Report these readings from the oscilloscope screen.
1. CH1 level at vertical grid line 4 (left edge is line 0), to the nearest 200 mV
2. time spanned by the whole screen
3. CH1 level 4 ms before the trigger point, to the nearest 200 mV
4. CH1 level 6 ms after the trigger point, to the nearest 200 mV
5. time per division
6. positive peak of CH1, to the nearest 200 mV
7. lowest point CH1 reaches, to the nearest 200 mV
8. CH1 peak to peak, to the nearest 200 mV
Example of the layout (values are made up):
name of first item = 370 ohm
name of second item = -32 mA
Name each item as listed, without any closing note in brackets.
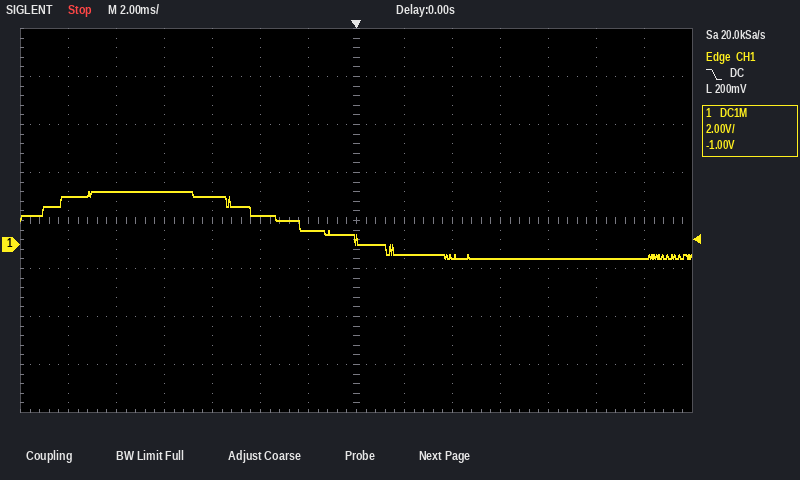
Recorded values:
CH1 level at vertical grid line 4 (left edge is line 0), to the nearest 200 mV = 2.0 V
time spanned by the whole screen = 28 ms
CH1 level 4 ms before the trigger point, to the nearest 200 mV = 1.2 V
CH1 level 6 ms after the trigger point, to the nearest 200 mV = -600 mV
time per division = 2 ms
positive peak of CH1, to the nearest 200 mV = 2.2 V
lowest point CH1 reaches, to the nearest 200 mV = -600 mV
CH1 peak to peak, to the nearest 200 mV = 2.8 V
